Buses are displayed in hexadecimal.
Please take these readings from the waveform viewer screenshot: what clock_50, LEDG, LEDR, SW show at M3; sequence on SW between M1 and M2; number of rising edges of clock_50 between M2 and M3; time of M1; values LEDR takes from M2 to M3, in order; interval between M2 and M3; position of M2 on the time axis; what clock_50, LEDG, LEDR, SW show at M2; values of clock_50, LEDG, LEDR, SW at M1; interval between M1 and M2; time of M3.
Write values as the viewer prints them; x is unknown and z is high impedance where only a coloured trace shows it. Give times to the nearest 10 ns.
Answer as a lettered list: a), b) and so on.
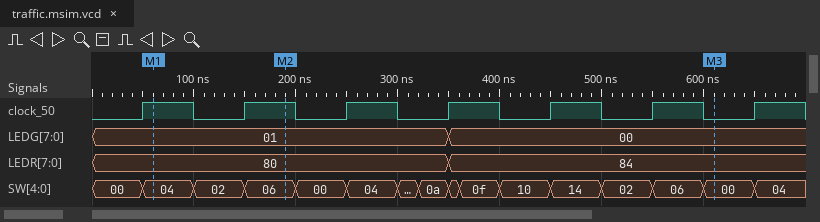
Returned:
a) clock_50=0, LEDG=00, LEDR=84, SW=00
b) 04, 02, 06
c) 4
d) 60 ns
e) 80, 84
f) 420 ns
g) 190 ns
h) clock_50=1, LEDG=01, LEDR=80, SW=06
i) clock_50=1, LEDG=01, LEDR=80, SW=04
j) 130 ns
k) 610 ns
